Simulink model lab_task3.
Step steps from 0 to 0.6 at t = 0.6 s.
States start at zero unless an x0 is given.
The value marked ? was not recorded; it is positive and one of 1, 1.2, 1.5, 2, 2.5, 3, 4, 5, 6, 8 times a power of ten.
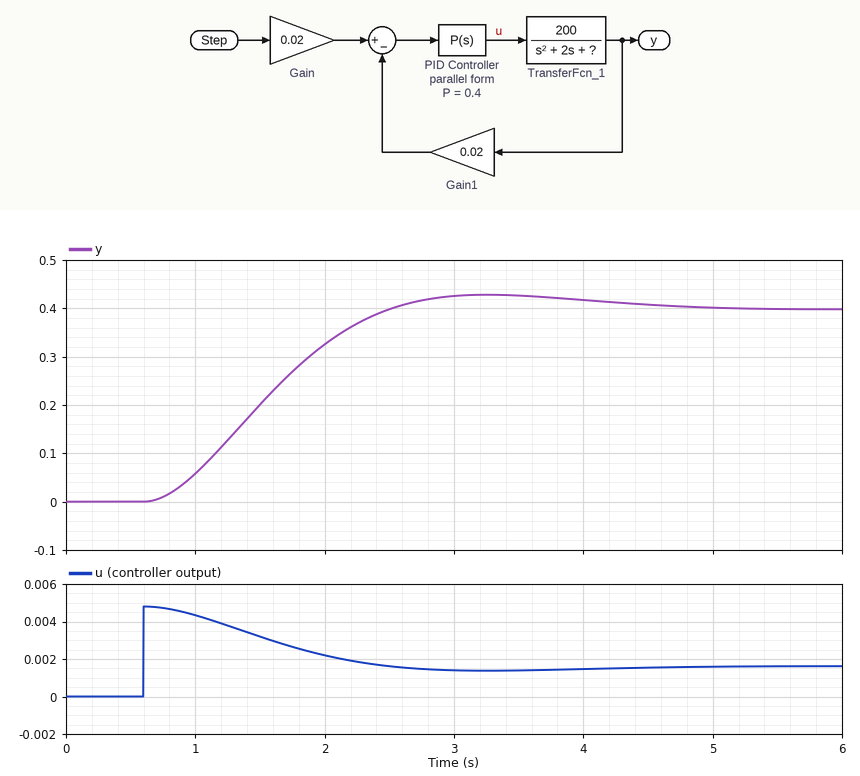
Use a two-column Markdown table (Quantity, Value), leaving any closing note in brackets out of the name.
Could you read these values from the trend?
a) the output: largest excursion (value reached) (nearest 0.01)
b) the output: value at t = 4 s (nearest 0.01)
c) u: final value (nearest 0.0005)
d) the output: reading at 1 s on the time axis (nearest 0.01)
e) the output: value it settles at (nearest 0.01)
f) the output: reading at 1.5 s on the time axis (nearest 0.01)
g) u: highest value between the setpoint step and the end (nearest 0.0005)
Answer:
| Quantity | Value |
|---|---|
| the output: largest excursion (value reached) | 0.43 |
| the output: value at t = 4 s | 0.42 |
| u: final value | 0.0015 |
| the output: reading at 1 s on the time axis | 0.06 |
| the output: value it settles at | 0.40 |
| the output: reading at 1.5 s on the time axis | 0.20 |
| u: highest value between the setpoint step and the end | 0.0050 |
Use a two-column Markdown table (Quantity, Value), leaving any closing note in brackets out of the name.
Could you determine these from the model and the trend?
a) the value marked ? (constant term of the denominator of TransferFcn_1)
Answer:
| Quantity | Value |
|---|---|
| the value marked ? | 0.8 |
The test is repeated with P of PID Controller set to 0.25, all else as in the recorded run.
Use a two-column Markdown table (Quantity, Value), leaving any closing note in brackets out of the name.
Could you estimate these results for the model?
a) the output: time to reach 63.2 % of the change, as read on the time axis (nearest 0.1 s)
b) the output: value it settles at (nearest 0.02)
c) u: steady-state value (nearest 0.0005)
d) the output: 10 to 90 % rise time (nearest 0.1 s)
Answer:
| Quantity | Value |
|---|---|
| the output: time to reach 63.2 % of the change, as read on the time axis | 1.9 s |
| the output: value it settles at | 0.34 |
| u: steady-state value | 0.0015 |
| the output: 10 to 90 % rise time | 1.7 s |
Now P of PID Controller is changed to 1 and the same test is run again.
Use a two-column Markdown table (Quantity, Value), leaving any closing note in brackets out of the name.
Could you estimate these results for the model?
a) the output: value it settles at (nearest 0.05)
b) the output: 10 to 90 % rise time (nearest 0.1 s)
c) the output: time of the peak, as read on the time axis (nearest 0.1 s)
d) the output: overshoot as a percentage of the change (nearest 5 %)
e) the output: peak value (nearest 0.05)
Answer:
| Quantity | Value |
|---|---|
| the output: value it settles at | 0.50 |
| the output: 10 to 90 % rise time | 0.7 s |
| the output: time of the peak, as read on the time axis | 2.2 s |
| the output: overshoot as a percentage of the change | 20 % |
| the output: peak value | 0.60 |
